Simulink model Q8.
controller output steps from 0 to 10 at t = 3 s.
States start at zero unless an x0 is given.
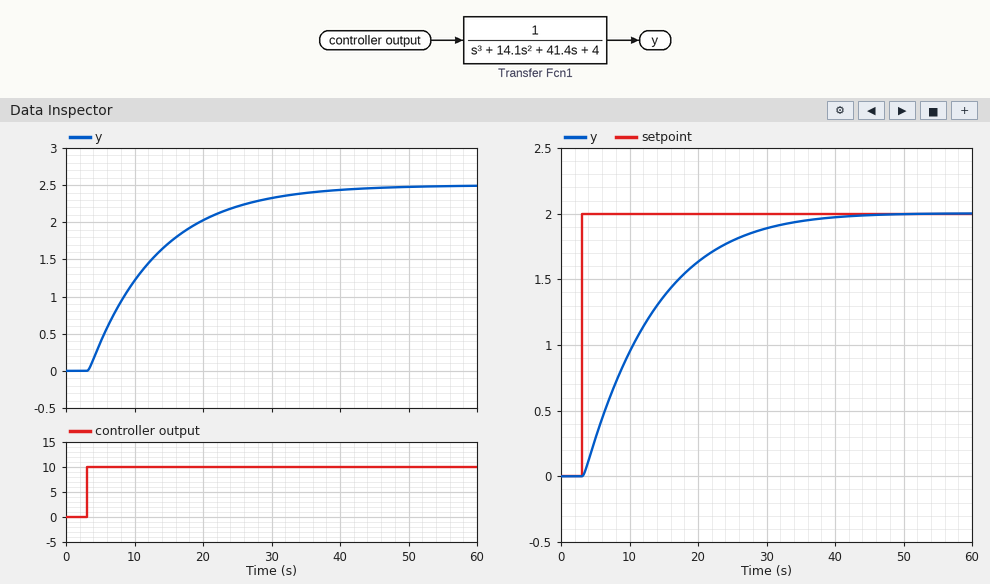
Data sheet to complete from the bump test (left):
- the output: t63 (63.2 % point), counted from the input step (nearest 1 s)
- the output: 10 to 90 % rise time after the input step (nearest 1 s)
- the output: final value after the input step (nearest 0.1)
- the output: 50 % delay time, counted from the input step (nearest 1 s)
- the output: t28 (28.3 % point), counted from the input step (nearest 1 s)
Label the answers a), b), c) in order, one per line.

a) 10 s
b) 22 s
c) 2.5
d) 7 s
e) 4 s
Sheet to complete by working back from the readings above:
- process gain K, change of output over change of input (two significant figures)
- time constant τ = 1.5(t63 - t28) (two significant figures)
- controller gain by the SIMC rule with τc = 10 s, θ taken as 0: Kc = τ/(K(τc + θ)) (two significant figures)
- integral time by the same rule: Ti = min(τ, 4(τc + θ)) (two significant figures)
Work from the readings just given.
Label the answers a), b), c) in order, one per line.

a) 0.25
b) 9.0 s
c) 3.6
d) 9.0 s
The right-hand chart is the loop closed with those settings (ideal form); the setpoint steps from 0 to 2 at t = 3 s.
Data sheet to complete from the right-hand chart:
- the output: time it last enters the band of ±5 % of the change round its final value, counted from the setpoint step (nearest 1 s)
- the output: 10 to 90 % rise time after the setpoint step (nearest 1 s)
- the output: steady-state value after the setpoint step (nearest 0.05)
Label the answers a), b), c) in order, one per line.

a) 28 s
b) 21 s
c) 2.00
